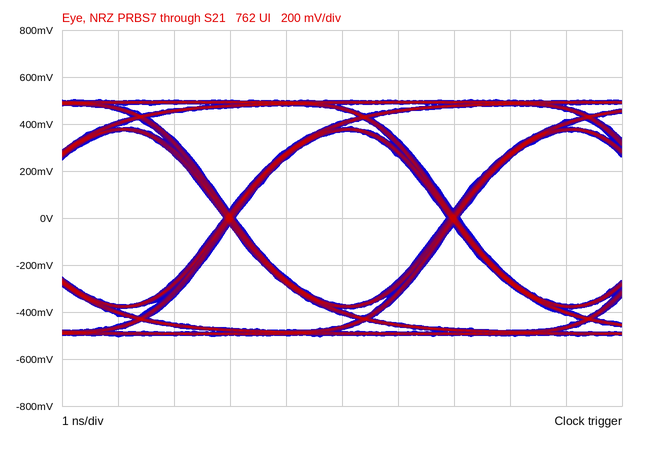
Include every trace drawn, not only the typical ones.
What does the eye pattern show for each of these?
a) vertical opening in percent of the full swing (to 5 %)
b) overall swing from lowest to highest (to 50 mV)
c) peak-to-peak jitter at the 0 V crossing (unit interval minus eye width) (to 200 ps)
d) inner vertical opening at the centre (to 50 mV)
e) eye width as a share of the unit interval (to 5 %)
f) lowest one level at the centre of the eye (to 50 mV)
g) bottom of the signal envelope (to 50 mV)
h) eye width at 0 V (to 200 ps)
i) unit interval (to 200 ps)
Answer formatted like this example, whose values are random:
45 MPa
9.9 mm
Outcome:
75 %
1.00 V
200 ps
750 mV
95 %
350 mV
-500 mV
3.8 ns
4.0 ns
